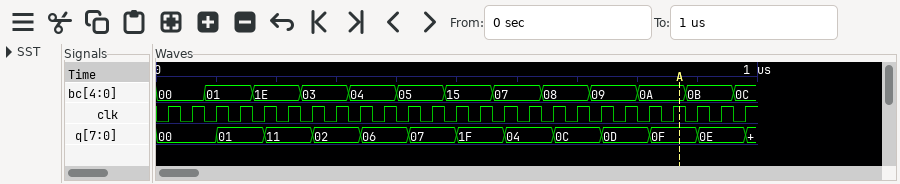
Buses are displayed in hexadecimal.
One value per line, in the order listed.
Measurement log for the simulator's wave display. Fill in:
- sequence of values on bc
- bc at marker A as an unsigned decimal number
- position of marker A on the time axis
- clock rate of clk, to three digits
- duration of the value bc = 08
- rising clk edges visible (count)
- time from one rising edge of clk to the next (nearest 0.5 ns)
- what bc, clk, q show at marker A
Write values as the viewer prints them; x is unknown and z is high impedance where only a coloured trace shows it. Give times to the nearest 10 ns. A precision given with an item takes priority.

00, 01, 1E, 03, 04, 05, 15, 07, 08, 09, 0A, 0B, 0C
10
870 ns
25.0 MHz
80 ns
25
40 ns
bc=0A, clk=1, q=0F
